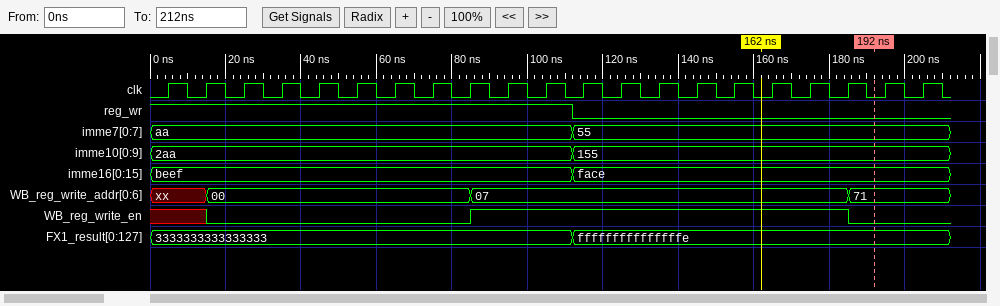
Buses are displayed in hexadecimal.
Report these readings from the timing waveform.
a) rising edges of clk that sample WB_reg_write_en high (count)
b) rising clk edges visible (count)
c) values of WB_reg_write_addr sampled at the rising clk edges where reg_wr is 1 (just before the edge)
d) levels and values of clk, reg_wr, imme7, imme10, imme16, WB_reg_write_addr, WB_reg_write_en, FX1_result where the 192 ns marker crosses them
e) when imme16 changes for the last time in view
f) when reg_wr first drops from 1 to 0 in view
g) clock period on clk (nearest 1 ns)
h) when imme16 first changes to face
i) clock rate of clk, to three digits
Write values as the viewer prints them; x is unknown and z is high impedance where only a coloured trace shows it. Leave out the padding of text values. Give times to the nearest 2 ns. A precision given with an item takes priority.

10
21
xx, xx, 00, 00, 00, 00, 00, 00, 00, 07, 07
clk=0, reg_wr=0, imme7=55, imme10=155, imme16=face, WB_reg_write_addr=71, WB_reg_write_en=0, FX1_result=fffffffffffffffe
112 ns
112 ns
10 ns
112 ns
100 MHz
